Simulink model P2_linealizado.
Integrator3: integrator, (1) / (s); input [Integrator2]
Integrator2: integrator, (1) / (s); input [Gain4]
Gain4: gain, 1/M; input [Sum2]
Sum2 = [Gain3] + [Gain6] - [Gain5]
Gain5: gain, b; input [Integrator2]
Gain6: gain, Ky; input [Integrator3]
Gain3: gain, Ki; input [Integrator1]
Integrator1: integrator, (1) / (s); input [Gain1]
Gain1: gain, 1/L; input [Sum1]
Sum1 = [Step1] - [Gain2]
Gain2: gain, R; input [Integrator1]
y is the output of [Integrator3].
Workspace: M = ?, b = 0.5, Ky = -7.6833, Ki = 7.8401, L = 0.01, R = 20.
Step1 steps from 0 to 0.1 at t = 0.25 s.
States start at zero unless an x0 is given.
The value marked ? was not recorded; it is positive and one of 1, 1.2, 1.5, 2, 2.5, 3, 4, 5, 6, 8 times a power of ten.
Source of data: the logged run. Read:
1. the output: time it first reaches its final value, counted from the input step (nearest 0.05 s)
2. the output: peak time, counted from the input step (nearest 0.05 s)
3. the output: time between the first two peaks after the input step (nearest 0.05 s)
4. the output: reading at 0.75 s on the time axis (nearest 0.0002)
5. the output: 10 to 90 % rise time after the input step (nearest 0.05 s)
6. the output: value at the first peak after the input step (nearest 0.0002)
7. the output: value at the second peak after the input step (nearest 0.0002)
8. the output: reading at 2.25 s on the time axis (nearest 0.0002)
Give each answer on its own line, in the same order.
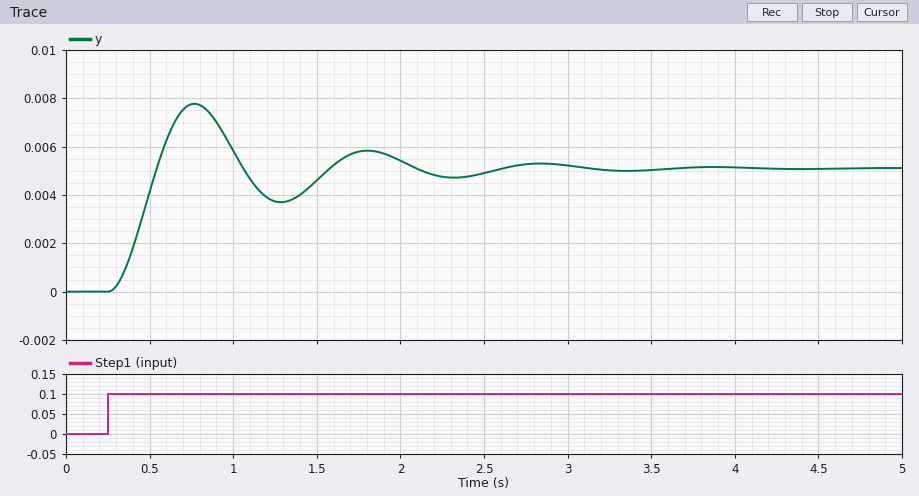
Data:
0.30 s
0.50 s
1.05 s
0.0078
0.20 s
0.0078
0.0058
0.0048
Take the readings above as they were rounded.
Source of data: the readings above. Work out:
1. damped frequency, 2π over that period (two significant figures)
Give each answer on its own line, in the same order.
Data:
6.0 rad/s
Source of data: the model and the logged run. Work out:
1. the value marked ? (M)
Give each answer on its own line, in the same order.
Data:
0.2
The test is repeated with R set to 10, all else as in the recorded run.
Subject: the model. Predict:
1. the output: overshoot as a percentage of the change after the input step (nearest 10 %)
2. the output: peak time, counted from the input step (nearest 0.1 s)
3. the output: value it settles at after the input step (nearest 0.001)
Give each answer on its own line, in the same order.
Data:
50 %
0.5 s
0.010
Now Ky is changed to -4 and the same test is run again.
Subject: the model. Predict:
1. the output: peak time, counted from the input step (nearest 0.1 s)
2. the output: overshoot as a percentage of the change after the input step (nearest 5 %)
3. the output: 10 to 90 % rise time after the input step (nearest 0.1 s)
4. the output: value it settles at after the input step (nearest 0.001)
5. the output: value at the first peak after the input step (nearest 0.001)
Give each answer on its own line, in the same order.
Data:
0.7 s
40 %
0.3 s
0.010
0.014
